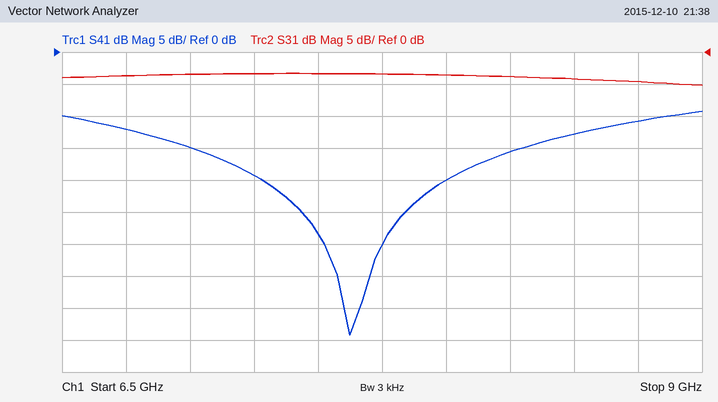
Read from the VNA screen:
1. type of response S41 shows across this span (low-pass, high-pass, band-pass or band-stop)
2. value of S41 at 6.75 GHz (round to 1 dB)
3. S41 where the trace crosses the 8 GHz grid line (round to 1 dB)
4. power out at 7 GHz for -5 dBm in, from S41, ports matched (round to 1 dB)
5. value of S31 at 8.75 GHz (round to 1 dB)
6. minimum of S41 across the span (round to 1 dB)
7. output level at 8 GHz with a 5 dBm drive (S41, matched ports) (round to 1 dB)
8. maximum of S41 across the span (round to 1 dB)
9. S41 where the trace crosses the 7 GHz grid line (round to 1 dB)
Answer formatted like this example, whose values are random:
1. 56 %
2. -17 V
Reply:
1. band-stop
2. -12 dB
3. -20 dB
4. -20 dBm
5. -5 dB
6. -44 dB
7. -15 dBm
8. -9 dB
9. -15 dB
